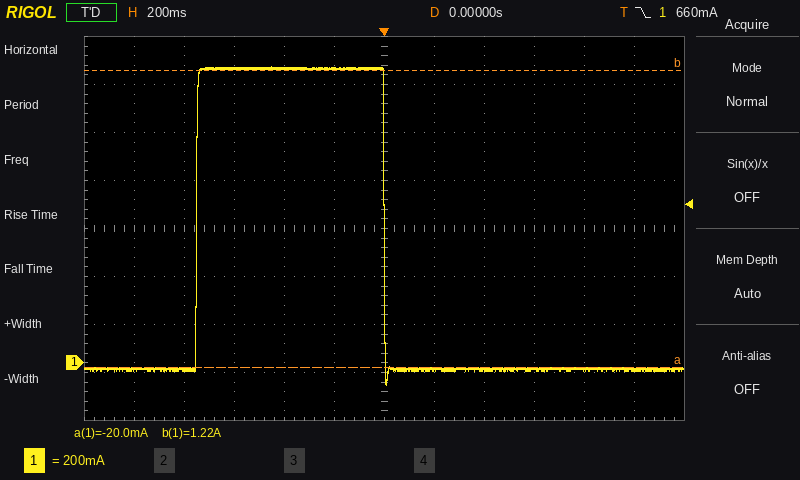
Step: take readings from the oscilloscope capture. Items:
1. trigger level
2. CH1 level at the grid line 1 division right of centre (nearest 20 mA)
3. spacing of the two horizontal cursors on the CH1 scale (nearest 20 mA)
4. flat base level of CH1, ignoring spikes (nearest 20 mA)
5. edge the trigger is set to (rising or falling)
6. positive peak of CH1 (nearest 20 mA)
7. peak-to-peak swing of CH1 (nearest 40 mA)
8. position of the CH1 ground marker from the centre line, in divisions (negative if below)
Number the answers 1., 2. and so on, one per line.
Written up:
1. 660 mA
2. -20 mA
3. 1.24 A
4. -20 mA
5. falling
6. 1.24 A
7. 1.32 A
8. -2.8 div
